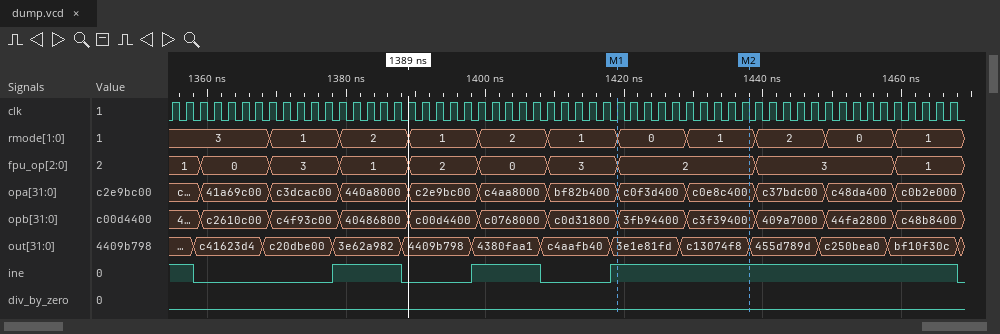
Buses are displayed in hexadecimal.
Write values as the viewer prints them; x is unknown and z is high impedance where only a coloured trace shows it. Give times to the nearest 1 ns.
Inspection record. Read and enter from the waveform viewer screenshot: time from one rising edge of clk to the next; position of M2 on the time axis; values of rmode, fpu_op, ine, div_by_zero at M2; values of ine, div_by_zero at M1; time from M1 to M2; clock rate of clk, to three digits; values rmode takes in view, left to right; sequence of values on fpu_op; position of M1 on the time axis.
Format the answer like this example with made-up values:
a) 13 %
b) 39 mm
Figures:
a) 2 ns
b) 1438 ns
c) rmode=1, fpu_op=2, ine=1, div_by_zero=0
d) ine=1, div_by_zero=0
e) 19 ns
f) 500 MHz
g) 3, 1, 2, 1, 2, 1, 0, 1, 2, 0, 1
h) 1, 0, 3, 1, 2, 0, 3, 2, 3, 1
i) 1419 ns
